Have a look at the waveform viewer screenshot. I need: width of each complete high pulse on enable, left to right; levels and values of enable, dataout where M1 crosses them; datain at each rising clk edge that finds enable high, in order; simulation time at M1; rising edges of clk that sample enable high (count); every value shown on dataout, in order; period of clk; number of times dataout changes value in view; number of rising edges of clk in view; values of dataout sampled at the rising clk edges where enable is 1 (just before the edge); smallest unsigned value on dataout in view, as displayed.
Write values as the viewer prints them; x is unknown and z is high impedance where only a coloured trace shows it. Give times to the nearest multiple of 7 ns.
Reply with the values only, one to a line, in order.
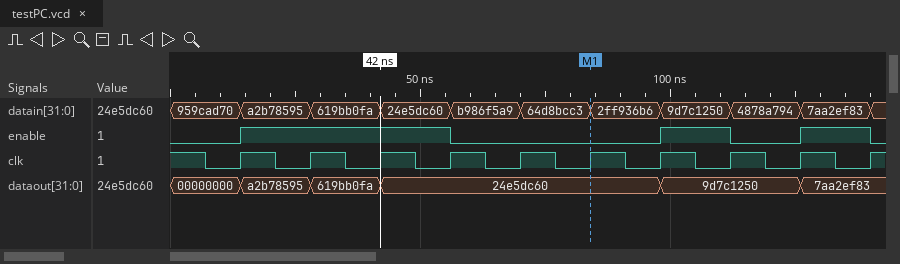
42 ns, 14 ns, 14 ns
enable=0, dataout=24e5dc60
a2b78595, 619bb0fa, 24e5dc60, 9d7c1250, 7aa2ef83
84 ns
5
00000000, a2b78595, 619bb0fa, 24e5dc60, 9d7c1250, 7aa2ef83
14 ns
5
10
a2b78595, 619bb0fa, 24e5dc60, 9d7c1250, 7aa2ef83
00000000
